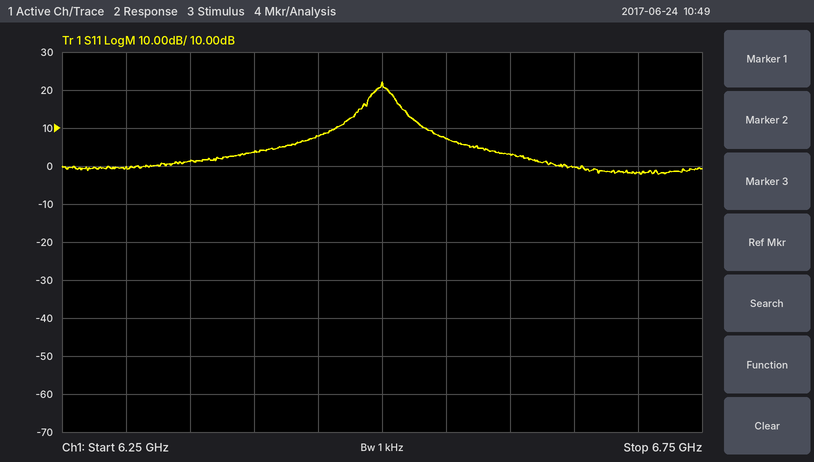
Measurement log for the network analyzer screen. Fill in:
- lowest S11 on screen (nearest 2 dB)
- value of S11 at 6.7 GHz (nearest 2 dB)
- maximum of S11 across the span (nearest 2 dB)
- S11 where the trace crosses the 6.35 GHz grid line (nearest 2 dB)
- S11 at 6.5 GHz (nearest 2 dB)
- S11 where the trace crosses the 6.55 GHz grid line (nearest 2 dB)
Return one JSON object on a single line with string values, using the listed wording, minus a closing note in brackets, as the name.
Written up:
{"lowest S11 on screen": "-2 dB", "value of S11 at 6.7 GHz": "-2 dB", "maximum of S11 across the span": "22 dB", "S11 where the trace crosses the 6.35 GHz grid line": "2 dB", "S11 at 6.5 GHz": "22 dB", "S11 where the trace crosses the 6.55 GHz grid line": "8 dB"}
